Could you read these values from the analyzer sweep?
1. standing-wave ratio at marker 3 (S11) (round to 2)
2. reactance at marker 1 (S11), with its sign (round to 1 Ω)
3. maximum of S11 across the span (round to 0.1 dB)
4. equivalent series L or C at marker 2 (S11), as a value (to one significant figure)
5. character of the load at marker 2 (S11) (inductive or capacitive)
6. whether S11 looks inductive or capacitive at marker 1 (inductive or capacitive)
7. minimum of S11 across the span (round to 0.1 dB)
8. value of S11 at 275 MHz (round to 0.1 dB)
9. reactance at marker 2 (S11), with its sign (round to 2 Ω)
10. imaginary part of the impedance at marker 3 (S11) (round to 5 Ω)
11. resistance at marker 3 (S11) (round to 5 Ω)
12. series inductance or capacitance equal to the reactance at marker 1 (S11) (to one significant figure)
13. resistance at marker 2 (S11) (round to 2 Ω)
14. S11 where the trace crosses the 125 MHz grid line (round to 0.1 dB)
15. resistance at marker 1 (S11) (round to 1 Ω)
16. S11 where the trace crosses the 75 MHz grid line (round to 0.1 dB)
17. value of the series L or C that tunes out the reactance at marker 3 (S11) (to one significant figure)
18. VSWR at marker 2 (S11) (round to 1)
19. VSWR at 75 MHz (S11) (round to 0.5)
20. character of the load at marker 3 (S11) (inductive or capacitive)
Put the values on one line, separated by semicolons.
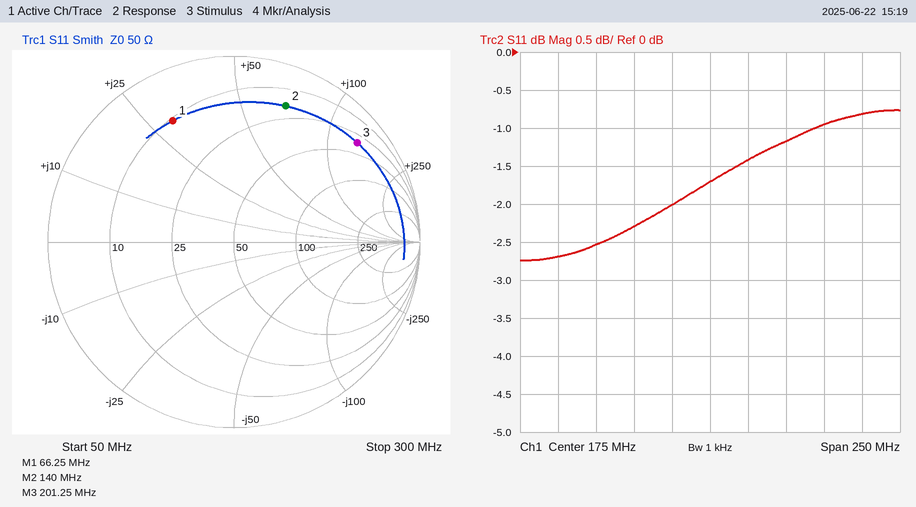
12; +30 Ω; -0.8 dB; 80 nH; inductive; inductive; -2.7 dB; -0.8 dB; +70 Ω; +135 Ω; 35 Ω; 70 nH; 18 Ω; -2.3 dB; 11 Ω; -2.7 dB; 6 pF; 8; 6.5; inductive
